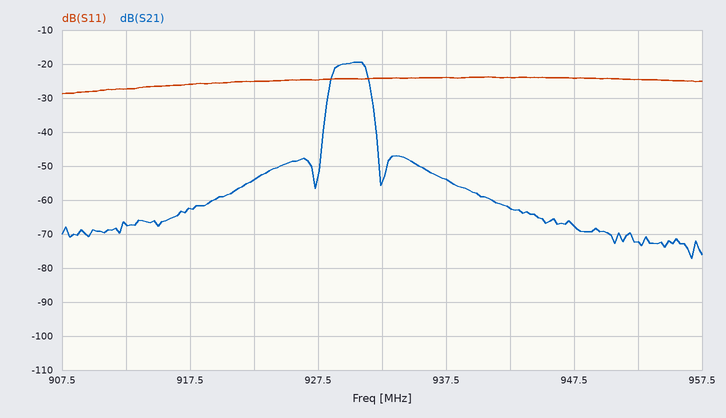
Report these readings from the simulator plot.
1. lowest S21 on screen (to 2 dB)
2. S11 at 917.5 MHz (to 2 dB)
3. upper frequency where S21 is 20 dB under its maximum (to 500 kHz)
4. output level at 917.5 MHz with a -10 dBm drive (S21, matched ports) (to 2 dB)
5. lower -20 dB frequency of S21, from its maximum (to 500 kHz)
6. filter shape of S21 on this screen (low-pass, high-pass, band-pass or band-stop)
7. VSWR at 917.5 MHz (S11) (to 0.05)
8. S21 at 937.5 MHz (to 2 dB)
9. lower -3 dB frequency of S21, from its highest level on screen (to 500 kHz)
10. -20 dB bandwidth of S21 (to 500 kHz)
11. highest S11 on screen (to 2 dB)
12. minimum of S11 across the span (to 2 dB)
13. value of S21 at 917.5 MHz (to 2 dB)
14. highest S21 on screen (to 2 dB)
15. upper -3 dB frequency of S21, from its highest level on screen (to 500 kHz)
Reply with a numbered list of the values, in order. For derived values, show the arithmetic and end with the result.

1. -78 dB
2. -26 dB
3. 932.0 MHz
4. -10 dBm + (-62 dB) = -72 dBm
5. 928.0 MHz
6. band-pass
7. |Γ| = 10^(-26/20) = 0.0501; VSWR = (1 + 0.0501)/(1 − 0.0501) ≈ 1.11, so 1.10 to the nearest 0.05
8. -54 dB
9. 928.5 MHz
10. 932.0 MHz − 928.0 MHz = 4.0 MHz
11. -24 dB
12. -28 dB
13. -62 dB
14. -20 dB
15. 931.5 MHz
